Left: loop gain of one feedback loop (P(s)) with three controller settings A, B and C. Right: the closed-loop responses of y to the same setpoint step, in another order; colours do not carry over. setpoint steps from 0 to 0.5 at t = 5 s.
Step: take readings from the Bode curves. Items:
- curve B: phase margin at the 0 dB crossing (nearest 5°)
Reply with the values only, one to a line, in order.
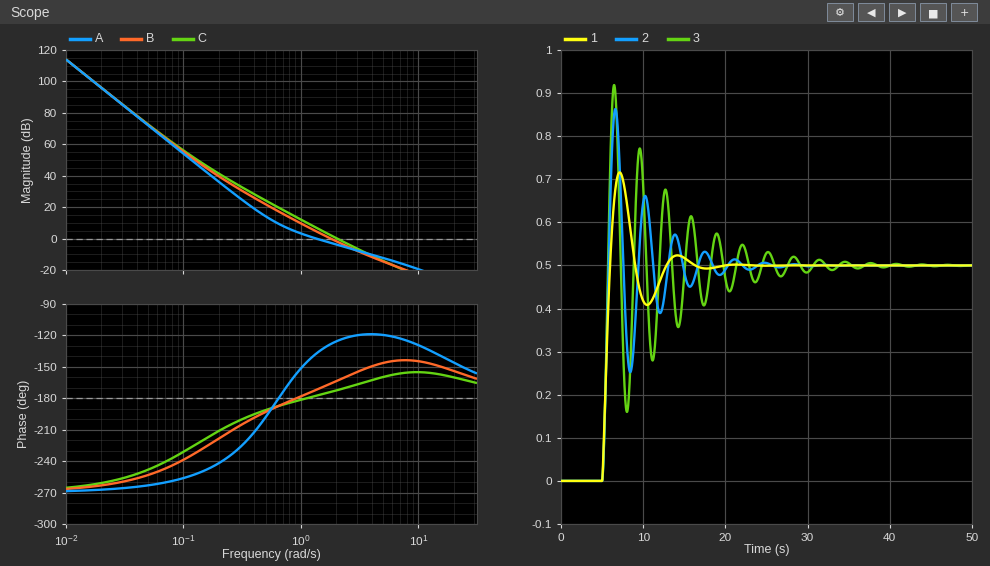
15°
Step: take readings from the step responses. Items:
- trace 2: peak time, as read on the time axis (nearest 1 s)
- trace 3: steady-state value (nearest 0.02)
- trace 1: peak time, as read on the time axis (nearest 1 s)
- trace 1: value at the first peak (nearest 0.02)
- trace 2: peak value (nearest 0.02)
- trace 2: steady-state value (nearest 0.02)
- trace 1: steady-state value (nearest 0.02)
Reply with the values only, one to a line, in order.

7 s
0.50
7 s
0.72
0.86
0.50
0.50
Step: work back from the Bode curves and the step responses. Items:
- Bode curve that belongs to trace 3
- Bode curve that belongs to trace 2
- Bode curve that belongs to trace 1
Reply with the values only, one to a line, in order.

C
B
A
